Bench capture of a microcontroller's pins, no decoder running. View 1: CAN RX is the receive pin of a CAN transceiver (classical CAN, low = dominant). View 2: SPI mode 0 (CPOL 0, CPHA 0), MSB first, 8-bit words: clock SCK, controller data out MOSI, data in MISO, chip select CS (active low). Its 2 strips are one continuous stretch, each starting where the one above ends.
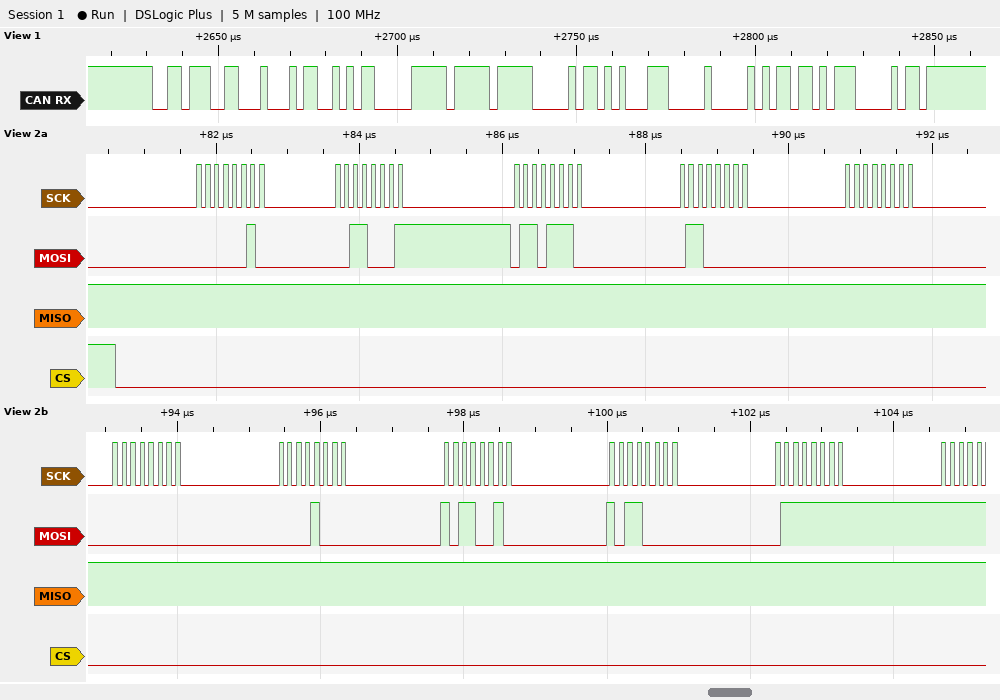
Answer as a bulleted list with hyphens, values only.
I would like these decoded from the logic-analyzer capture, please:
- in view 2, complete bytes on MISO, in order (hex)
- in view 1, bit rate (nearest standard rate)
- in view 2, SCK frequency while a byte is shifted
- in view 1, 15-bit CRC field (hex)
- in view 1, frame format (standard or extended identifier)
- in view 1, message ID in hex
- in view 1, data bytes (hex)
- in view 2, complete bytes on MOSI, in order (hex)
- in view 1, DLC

- 0xFF 0xFF 0xFF 0xFF 0xFF 0xFF 0xFF 0xFF 0xFF 0xFF
- 500 kbit/s
- 8 MHz
- 0x6B81
- standard
- 0x373
- B2 B0 7F FE 0D 47 00 16
- 0x02 0x31 0x6E 0x60 0x00 0x00 0x08 0xB2 0xB0 0x7F
- 8
